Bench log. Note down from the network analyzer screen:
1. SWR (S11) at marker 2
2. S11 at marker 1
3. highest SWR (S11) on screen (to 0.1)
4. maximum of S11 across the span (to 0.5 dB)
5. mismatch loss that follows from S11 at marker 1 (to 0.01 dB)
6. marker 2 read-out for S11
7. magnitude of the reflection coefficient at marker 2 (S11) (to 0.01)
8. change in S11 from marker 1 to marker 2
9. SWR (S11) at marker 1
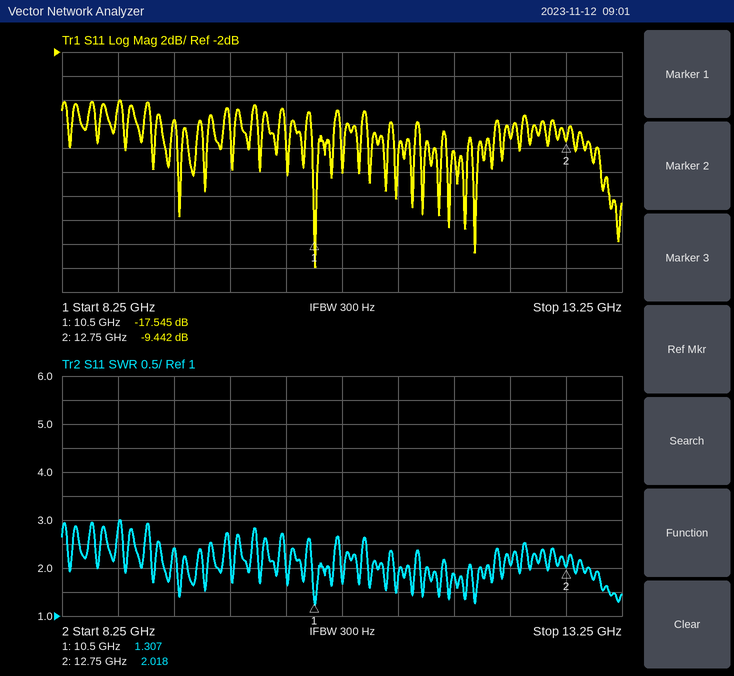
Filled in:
2.018
-17.545 dB
3.0
-6.0 dB
0.08 dB
-9.442 dB
0.34
8.103 dB
1.307
